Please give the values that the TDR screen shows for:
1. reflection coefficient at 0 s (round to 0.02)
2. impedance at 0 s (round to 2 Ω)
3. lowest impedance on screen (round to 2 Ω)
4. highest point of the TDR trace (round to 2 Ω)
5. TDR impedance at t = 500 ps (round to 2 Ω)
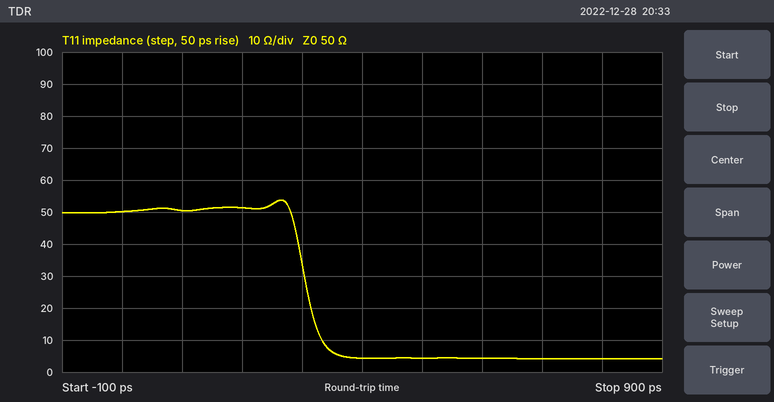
0.00
50 Ω
4 Ω
54 Ω
4 Ω
